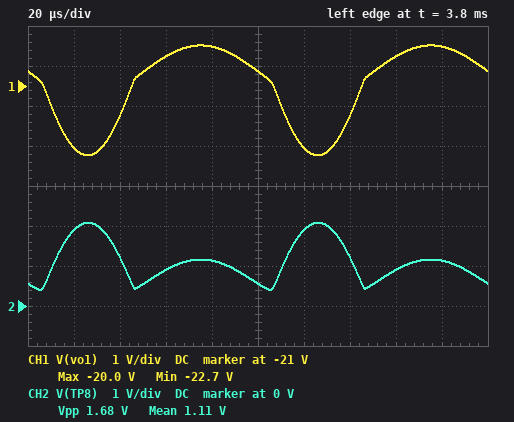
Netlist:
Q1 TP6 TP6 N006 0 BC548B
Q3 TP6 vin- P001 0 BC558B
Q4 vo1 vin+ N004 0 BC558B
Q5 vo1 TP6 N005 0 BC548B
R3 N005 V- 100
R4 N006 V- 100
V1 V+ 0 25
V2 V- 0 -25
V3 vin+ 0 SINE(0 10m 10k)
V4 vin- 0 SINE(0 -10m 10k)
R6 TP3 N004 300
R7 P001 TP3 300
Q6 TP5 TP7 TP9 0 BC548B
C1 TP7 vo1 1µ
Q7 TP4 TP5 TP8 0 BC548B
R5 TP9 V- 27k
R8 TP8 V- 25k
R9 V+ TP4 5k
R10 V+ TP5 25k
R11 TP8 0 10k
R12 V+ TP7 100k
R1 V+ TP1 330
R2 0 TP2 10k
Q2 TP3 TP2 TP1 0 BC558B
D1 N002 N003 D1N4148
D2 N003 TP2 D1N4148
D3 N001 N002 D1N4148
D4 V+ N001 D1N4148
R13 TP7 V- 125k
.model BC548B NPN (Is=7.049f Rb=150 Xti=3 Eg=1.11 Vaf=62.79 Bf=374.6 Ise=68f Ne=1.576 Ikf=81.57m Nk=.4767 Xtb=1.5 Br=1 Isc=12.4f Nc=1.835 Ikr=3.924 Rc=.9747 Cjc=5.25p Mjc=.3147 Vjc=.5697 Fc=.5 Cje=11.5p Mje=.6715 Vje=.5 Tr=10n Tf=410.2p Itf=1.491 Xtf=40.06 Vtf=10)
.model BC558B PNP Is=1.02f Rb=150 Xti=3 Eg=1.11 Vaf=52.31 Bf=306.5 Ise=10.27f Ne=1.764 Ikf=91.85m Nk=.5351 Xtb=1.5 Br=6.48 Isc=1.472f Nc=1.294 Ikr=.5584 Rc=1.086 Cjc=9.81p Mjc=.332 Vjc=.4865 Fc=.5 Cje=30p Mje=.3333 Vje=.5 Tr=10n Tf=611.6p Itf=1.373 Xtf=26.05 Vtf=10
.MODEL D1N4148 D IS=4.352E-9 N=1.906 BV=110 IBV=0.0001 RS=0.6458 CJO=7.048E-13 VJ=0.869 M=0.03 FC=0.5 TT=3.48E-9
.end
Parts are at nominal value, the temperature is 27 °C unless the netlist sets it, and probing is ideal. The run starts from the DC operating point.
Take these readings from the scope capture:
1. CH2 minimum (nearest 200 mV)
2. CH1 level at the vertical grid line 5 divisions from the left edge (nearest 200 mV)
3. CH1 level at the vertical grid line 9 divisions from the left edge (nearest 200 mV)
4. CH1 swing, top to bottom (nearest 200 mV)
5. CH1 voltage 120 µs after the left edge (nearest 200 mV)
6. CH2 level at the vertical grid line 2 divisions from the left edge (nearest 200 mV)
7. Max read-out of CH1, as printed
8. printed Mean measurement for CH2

400 mV
-20.6 V
-20.0 V
2.8 V
-22.6 V
1.2 V
-20.0 V
1.11 V
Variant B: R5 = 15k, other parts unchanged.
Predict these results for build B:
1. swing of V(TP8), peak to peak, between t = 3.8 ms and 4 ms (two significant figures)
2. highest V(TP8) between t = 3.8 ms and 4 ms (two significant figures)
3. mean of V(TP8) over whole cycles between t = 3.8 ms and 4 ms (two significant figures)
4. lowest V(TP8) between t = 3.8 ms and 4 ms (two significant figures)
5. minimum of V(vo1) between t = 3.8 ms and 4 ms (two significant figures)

950 mV
-5.1 V
-5.6 V
-6.1 V
-21 V
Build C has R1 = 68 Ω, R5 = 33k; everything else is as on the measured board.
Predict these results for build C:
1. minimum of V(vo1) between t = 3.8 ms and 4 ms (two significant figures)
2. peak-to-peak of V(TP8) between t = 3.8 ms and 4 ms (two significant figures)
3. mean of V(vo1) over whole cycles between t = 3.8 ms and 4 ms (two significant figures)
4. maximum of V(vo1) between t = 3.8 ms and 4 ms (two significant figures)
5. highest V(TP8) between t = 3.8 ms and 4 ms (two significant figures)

-15 V
2.9 V
-13 V
-11 V
5.7 V
